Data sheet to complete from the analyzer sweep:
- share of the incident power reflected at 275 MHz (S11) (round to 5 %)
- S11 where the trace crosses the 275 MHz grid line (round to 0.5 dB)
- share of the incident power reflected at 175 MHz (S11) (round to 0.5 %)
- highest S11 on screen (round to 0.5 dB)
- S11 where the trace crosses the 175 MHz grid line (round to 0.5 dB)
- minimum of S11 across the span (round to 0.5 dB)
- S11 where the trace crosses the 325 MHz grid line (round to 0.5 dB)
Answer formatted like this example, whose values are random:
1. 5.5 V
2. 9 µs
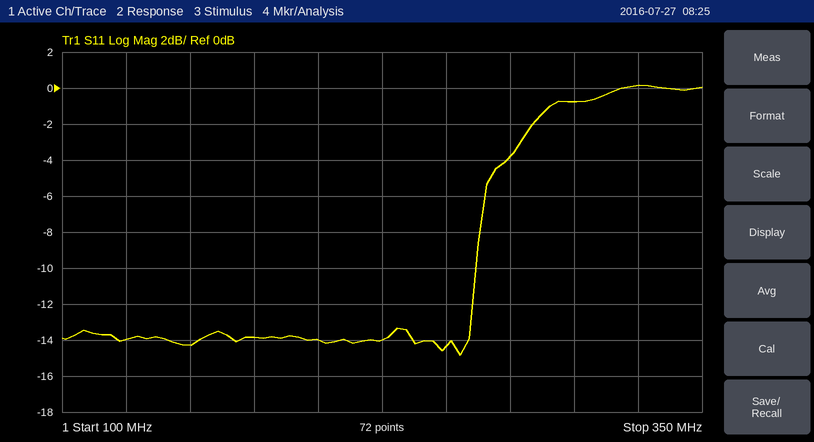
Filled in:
1. 40 %
2. -4.0 dB
3. 4.0 %
4. 0.0 dB
5. -14.0 dB
6. -15.0 dB
7. 0.0 dB
